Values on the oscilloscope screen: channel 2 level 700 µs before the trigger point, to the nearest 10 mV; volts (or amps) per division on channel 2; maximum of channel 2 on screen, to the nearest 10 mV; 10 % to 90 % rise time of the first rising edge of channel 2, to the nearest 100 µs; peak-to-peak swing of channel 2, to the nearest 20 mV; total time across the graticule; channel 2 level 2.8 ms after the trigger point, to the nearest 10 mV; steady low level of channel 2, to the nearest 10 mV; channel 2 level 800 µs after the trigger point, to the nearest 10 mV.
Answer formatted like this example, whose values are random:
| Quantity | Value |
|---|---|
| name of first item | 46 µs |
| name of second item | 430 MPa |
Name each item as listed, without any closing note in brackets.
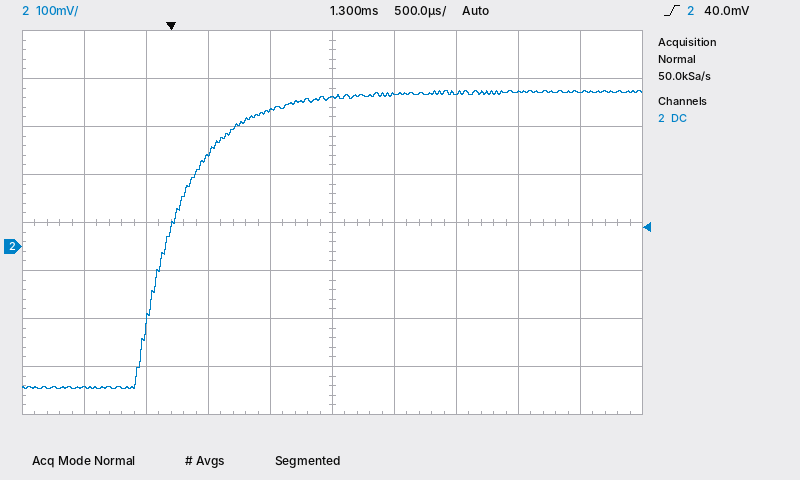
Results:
| Quantity | Value |
|---|---|
| channel 2 level 700 µs before the trigger point, to the nearest 10 mV | -290 mV |
| volts (or amps) per division on channel 2 | 100 mV |
| maximum of channel 2 on screen, to the nearest 10 mV | 320 mV |
| 10 % to 90 % rise time of the first rising edge of channel 2, to the nearest 100 µs | 800 µs |
| peak-to-peak swing of channel 2, to the nearest 20 mV | 620 mV |
| total time across the graticule | 5 ms |
| channel 2 level 2.8 ms after the trigger point, to the nearest 10 mV | 320 mV |
| steady low level of channel 2, to the nearest 10 mV | -290 mV |
| channel 2 level 800 µs after the trigger point, to the nearest 10 mV | 280 mV |
